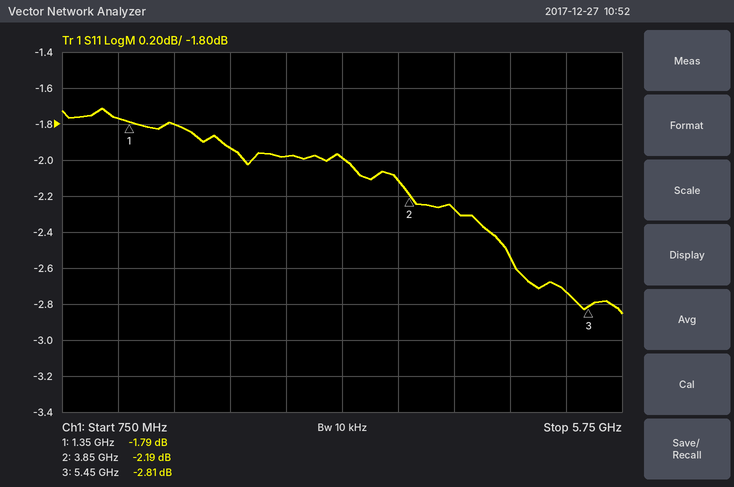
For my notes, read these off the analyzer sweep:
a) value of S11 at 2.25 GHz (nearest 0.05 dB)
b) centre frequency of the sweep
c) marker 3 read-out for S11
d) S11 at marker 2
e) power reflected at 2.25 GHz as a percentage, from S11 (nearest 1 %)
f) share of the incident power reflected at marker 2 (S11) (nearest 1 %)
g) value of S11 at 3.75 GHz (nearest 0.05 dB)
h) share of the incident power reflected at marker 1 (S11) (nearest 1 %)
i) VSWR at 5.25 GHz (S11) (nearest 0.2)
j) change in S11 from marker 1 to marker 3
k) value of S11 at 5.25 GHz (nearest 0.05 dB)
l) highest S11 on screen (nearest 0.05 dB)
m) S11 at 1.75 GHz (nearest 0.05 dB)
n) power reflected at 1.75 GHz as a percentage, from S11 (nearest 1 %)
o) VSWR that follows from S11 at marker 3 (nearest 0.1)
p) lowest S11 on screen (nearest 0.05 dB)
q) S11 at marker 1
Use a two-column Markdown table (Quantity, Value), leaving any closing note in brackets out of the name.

| Quantity | Value |
|---|---|
| value of S11 at 2.25 GHz | -1.95 dB |
| centre frequency of the sweep | 3.25 GHz |
| marker 3 read-out for S11 | -2.81 dB |
| S11 at marker 2 | -2.19 dB |
| power reflected at 2.25 GHz as a percentage, from S11 | 64 % |
| share of the incident power reflected at marker 2 (S11) | 60 % |
| value of S11 at 3.75 GHz | -2.10 dB |
| share of the incident power reflected at marker 1 (S11) | 66 % |
| VSWR at 5.25 GHz (S11) | 6.4 |
| change in S11 from marker 1 to marker 3 | -1.02 dB |
| value of S11 at 5.25 GHz | -2.75 dB |
| highest S11 on screen | -1.70 dB |
| S11 at 1.75 GHz | -1.80 dB |
| power reflected at 1.75 GHz as a percentage, from S11 | 66 % |
| VSWR that follows from S11 at marker 3 | 6.2 |
| lowest S11 on screen | -2.85 dB |
| S11 at marker 1 | -1.79 dB |
